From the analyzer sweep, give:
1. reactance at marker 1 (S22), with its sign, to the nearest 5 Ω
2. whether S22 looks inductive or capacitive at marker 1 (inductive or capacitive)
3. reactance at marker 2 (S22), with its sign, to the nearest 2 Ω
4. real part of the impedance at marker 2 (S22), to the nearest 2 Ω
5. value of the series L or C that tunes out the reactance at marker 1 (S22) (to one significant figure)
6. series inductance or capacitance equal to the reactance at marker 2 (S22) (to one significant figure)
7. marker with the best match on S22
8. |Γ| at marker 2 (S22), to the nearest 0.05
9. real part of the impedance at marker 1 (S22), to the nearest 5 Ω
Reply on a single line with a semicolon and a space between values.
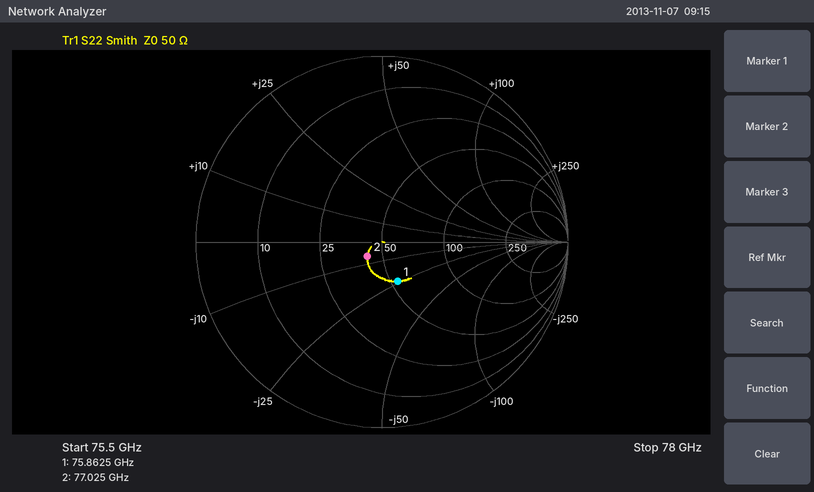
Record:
-25 Ω; capacitive; -6 Ω; 42 Ω; 50 pH; 300 fF; marker 2; 0.10; 55 Ω
